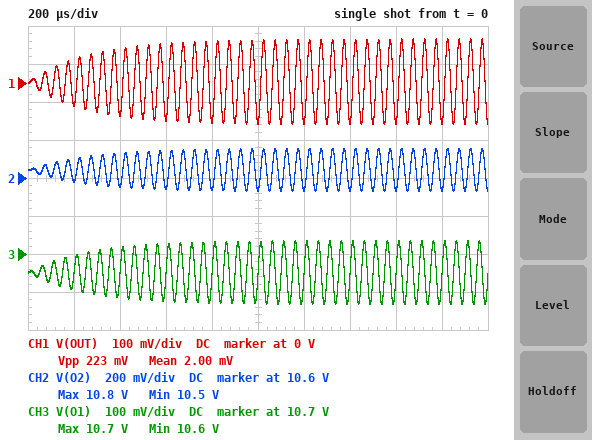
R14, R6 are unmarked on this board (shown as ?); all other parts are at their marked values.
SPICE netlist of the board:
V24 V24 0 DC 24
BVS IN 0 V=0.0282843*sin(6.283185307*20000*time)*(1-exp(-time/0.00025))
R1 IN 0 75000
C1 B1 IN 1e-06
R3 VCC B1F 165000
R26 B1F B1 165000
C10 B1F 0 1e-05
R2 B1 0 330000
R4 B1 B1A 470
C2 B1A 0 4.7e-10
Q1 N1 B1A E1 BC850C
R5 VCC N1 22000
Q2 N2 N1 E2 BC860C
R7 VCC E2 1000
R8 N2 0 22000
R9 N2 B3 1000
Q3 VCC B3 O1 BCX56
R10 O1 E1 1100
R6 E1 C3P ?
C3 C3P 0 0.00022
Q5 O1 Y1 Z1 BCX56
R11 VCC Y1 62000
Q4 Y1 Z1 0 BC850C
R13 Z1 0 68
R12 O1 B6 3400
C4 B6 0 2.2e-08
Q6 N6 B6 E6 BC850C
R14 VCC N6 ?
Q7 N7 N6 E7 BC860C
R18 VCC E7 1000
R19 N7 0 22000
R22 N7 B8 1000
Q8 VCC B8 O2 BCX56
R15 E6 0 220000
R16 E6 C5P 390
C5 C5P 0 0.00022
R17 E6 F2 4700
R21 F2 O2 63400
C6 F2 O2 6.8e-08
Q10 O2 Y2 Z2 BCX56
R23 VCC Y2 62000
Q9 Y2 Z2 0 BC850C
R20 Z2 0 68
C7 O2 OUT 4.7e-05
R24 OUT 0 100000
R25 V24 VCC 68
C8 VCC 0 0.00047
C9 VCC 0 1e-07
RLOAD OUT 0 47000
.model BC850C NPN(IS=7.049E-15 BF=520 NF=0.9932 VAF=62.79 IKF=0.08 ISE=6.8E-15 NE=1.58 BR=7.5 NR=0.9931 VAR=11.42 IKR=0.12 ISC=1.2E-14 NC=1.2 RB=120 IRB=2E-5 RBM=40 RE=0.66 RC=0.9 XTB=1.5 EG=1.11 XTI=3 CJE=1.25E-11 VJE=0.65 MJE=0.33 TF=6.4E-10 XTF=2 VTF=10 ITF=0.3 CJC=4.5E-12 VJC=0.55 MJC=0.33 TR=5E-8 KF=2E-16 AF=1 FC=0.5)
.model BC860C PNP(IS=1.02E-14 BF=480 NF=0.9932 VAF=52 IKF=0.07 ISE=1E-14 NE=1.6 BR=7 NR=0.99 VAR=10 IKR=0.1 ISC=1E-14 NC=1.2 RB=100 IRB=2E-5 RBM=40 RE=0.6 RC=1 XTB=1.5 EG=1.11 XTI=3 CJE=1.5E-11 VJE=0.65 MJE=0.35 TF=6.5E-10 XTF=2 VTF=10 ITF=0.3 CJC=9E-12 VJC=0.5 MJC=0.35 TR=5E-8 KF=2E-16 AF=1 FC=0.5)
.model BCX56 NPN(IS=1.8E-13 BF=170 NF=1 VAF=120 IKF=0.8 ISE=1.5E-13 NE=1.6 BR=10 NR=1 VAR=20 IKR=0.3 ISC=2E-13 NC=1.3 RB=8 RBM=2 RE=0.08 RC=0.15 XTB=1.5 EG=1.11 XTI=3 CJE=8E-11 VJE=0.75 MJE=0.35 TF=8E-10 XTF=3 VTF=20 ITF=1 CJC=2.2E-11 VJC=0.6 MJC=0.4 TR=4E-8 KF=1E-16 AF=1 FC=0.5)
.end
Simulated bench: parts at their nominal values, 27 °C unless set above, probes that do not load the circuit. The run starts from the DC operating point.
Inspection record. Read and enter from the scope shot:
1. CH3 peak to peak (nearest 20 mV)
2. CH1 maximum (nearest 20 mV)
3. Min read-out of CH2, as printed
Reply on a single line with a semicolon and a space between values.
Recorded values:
160 mV; 120 mV; 10.5 V
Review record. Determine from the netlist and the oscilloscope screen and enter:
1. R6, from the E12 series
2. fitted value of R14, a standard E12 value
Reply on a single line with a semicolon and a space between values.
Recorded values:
560 Ω; 33 kΩ
